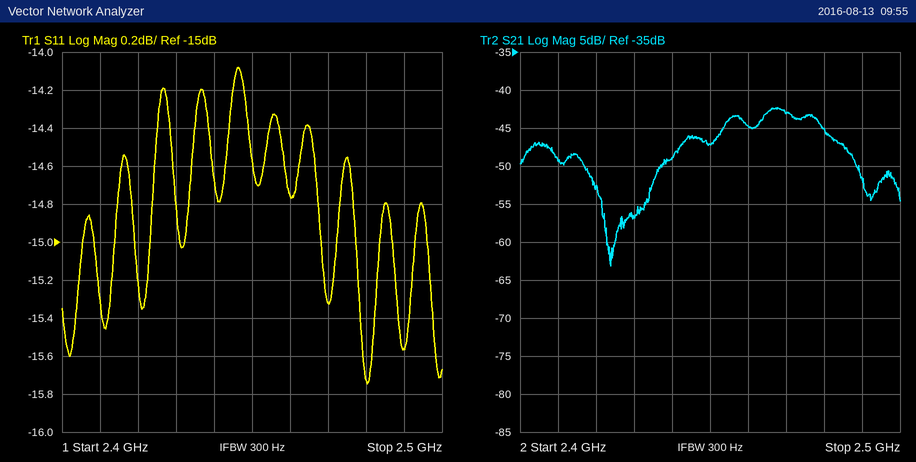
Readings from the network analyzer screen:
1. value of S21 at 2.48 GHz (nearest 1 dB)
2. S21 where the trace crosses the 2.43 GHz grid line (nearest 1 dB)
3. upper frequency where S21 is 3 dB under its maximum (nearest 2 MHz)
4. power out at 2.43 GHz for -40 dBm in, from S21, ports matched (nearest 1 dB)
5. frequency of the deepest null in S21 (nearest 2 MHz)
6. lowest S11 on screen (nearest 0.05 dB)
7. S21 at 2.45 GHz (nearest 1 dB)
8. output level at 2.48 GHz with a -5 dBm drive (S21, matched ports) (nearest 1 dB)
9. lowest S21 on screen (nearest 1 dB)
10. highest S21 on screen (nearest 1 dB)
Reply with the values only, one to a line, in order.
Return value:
-45 dB
-57 dB
2.480 GHz
-97 dBm
2.424 GHz
-15.75 dB
-47 dB
-50 dBm
-63 dB
-42 dB
